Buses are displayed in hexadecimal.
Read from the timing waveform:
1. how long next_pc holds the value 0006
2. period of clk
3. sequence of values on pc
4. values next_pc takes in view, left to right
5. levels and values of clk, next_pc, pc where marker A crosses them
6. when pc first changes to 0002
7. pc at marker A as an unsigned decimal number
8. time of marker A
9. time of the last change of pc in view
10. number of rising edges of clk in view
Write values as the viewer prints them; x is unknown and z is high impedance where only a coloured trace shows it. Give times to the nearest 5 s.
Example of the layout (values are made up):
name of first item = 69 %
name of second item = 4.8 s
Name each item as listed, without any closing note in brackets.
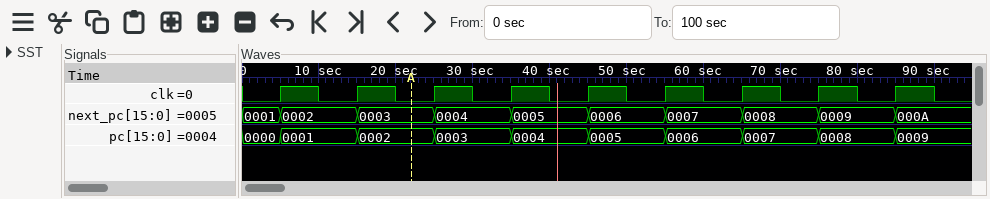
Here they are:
how long next_pc holds the value 0006 = 10 s
period of clk = 10 s
sequence of values on pc = 0000, 0001, 0002, 0003, 0004, 0005, 0006, 0007, 0008, 0009
values next_pc takes in view, left to right = 0001, 0002, 0003, 0004, 0005, 0006, 0007, 0008, 0009, 000A
levels and values of clk, next_pc, pc where marker A crosses them = clk=0, next_pc=0003, pc=0002
when pc first changes to 0002 = 15 s
pc at marker A as an unsigned decimal number = 2
time of marker A = 20 s
time of the last change of pc in view = 85 s
number of rising edges of clk in view = 9
